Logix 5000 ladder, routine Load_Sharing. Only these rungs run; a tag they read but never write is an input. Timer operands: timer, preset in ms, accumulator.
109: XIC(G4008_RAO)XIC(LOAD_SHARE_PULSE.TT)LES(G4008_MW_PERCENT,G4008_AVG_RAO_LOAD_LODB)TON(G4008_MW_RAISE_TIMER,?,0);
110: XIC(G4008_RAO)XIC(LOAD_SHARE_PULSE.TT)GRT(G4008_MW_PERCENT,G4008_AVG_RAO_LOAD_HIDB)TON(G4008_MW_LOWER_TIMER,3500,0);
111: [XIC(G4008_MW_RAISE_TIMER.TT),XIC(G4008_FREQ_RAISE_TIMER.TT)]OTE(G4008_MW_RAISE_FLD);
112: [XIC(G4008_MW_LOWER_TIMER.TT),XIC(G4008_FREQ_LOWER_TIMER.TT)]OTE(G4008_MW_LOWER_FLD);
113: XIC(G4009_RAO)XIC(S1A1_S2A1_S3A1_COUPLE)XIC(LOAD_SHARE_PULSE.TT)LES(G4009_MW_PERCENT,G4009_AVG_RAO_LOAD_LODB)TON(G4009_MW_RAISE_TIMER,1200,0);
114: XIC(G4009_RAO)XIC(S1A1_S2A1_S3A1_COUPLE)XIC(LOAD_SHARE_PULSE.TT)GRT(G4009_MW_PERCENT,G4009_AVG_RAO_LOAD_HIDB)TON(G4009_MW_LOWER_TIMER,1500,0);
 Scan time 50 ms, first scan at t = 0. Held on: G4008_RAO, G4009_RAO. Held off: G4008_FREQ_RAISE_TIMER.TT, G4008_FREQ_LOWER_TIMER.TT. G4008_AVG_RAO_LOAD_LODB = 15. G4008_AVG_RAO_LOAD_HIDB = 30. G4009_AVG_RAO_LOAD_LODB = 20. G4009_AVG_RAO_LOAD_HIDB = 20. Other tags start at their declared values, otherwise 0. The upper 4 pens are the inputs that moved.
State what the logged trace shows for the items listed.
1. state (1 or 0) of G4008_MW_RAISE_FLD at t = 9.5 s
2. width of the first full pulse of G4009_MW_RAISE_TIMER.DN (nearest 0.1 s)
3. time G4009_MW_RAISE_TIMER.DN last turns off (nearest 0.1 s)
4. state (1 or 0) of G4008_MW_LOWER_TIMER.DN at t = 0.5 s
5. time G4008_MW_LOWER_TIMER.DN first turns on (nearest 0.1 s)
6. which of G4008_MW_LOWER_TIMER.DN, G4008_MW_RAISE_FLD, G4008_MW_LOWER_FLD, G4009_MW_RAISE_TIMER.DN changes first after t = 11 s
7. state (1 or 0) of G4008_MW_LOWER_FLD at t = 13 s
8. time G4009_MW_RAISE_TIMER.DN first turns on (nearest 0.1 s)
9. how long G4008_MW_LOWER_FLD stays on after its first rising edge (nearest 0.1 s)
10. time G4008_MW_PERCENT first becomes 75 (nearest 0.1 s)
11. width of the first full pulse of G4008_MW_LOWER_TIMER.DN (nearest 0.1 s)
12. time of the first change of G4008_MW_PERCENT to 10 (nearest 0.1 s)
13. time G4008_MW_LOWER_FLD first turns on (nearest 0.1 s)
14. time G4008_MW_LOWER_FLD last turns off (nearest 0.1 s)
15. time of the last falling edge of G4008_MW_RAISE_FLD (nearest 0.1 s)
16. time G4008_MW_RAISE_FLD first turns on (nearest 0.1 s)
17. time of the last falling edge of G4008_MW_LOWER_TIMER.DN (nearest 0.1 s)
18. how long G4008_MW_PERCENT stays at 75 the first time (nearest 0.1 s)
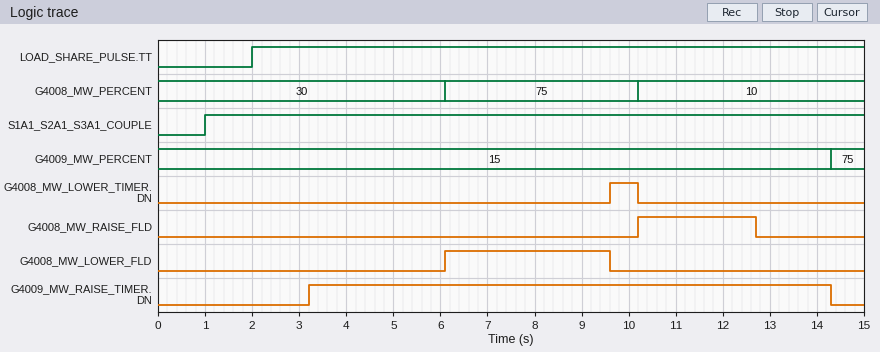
0
11.1 s
14.3 s
0
9.6 s
G4008_MW_RAISE_FLD
0
3.2 s
3.5 s
6.1 s
0.6 s
10.2 s
6.1 s
9.6 s
12.7 s
10.2 s
10.2 s
4.1 s
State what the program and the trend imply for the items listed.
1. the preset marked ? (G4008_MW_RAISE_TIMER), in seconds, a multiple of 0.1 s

2.5 s
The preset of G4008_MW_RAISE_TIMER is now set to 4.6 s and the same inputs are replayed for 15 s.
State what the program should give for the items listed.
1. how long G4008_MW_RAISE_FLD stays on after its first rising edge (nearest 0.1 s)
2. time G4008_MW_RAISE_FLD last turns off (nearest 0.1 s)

4.6 s
14.8 s
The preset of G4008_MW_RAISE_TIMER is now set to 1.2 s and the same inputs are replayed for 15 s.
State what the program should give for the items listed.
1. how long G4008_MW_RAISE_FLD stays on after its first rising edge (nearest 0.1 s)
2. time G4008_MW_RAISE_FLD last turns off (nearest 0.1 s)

1.2 s
11.4 s
